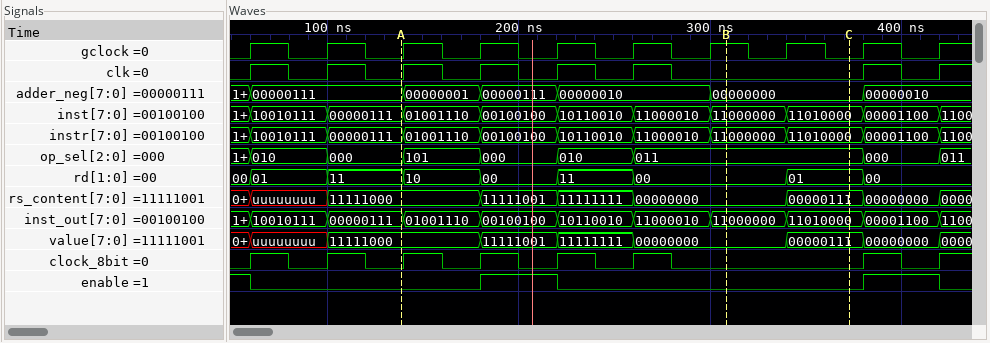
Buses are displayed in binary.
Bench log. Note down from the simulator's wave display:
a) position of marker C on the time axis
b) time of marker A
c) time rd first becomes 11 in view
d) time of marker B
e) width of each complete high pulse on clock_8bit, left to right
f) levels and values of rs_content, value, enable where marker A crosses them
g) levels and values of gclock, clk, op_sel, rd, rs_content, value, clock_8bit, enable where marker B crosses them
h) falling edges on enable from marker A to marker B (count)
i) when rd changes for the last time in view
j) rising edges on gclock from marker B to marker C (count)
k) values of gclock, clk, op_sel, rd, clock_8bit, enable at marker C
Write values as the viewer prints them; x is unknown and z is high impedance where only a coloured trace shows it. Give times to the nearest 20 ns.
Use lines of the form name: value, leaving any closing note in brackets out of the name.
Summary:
position of marker C on the time axis: 380 ns
time of marker A: 140 ns
time rd first becomes 11 in view: 100 ns
time of marker B: 300 ns
width of each complete high pulse on clock_8bit, left to right: 20 ns, 20 ns, 20 ns, 20 ns, 20 ns, 20 ns, 20 ns
levels and values of rs_content, value, enable where marker A crosses them: rs_content=11111000, value=11111000, enable=0
levels and values of gclock, clk, op_sel, rd, rs_content, value, clock_8bit, enable where marker B crosses them: gclock=1, clk=0, op_sel=011, rd=00, rs_content=00000000, value=00000000, clock_8bit=0, enable=0
falling edges on enable from marker A to marker B: 1
when rd changes for the last time in view: 380 ns
rising edges on gclock from marker B to marker C: 1
values of gclock, clk, op_sel, rd, clock_8bit, enable at marker C: gclock=0, clk=0, op_sel=011, rd=01, clock_8bit=0, enable=0
